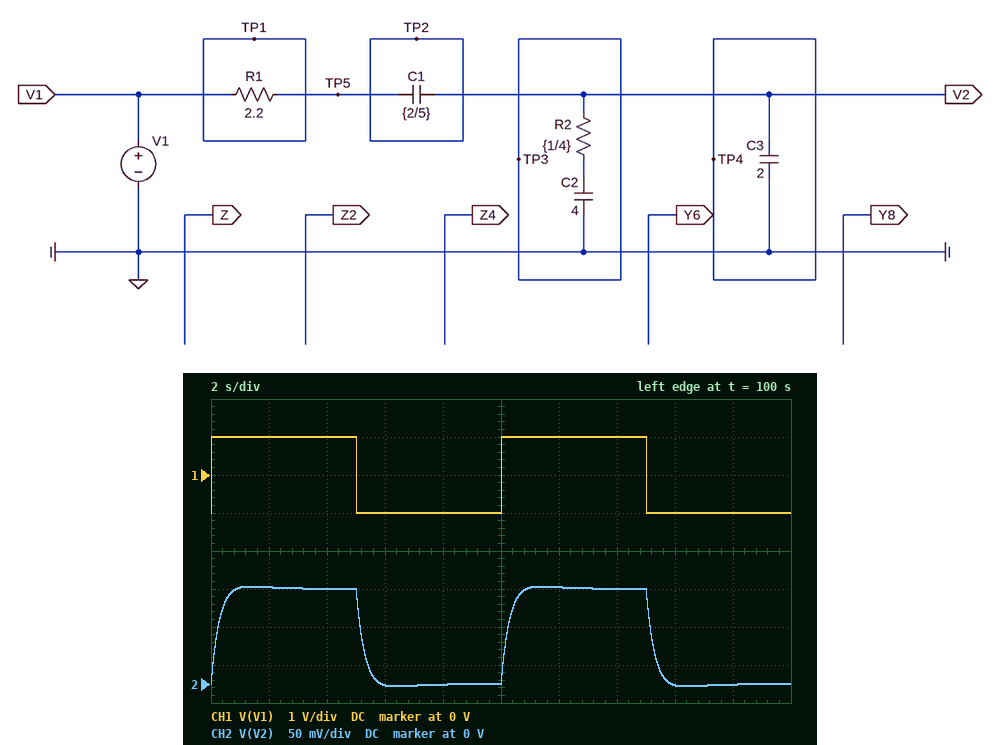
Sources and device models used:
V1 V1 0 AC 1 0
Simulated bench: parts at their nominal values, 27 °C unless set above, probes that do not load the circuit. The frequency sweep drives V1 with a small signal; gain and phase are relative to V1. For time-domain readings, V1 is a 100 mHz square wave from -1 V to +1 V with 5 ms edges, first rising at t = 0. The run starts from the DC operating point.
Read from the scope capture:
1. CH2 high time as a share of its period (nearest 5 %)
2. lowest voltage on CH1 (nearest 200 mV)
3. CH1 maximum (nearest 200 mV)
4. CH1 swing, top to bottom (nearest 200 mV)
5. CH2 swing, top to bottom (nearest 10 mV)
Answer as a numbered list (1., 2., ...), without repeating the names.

1. 50 %
2. -1.0 V
3. 1.0 V
4. 2.0 V
5. 130 mV
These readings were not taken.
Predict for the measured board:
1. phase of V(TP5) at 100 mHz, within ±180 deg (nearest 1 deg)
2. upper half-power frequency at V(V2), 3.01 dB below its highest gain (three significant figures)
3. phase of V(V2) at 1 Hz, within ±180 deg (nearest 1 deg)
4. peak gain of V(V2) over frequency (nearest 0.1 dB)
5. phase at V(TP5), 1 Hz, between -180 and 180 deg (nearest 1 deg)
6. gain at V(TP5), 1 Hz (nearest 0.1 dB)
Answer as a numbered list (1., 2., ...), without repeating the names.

1. -27 deg
2. 614 mHz
3. -62 deg
4. -24.0 dB
5. -76 deg
6. -13.7 dB
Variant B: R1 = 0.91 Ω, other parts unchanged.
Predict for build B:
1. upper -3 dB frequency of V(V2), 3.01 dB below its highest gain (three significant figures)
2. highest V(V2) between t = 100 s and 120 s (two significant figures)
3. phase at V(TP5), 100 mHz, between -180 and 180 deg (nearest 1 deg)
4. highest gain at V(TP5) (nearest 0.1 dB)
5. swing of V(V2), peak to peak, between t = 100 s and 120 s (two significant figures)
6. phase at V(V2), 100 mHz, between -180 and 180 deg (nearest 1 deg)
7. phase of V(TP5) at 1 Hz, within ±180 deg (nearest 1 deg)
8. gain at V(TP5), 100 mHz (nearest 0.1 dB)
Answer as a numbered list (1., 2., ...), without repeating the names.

1. 1.10 Hz
2. 170 mV
3. -12 deg
4. 0 dB
5. 220 mV
6. 7 deg
7. -61 deg
8. -0.2 dB
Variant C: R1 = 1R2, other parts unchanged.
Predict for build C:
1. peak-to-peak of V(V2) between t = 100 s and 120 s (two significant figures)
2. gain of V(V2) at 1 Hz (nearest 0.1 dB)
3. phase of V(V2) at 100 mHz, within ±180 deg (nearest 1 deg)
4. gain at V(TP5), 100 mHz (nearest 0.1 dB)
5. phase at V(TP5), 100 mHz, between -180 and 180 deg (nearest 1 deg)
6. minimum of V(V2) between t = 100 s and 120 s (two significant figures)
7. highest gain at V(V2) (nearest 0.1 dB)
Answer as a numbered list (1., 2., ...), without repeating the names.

1. 190 mV
2. -25.1 dB
3. 3 deg
4. -0.4 dB
5. -16 deg
6. -32 mV
7. -21.7 dB
